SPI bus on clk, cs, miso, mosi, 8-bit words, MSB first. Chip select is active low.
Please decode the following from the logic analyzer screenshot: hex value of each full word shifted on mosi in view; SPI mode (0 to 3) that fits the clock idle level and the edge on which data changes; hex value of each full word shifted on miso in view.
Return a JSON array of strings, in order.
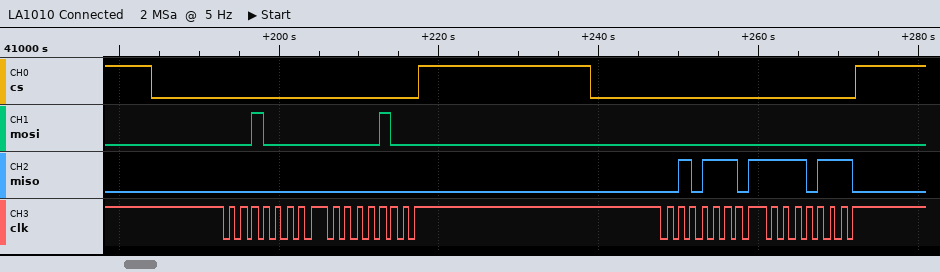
["10, 04, 00, 00", "2", "00, 00, 2E, F7"]
